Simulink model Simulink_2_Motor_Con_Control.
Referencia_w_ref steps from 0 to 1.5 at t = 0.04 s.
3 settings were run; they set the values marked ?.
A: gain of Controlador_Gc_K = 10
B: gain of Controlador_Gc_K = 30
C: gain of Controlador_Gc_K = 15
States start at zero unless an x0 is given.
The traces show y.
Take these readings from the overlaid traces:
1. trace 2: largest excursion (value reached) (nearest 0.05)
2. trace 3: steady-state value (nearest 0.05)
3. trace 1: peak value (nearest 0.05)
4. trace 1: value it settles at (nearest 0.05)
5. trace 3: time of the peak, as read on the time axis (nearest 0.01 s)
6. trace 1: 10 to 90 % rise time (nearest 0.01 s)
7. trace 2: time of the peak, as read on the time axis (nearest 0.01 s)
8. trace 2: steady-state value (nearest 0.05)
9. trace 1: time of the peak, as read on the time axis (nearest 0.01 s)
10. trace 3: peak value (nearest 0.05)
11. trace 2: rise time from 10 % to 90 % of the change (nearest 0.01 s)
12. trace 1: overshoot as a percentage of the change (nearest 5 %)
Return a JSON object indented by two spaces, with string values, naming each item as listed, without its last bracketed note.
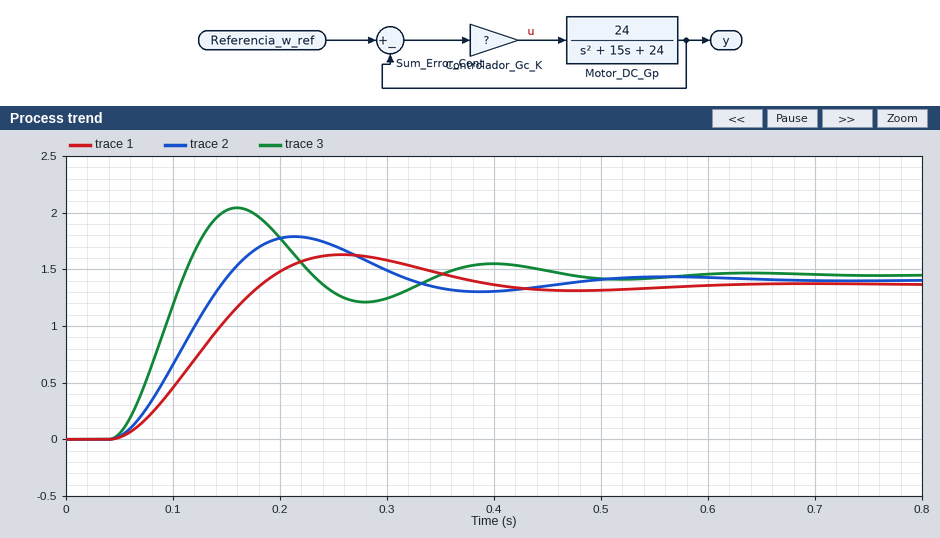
{
  "trace 2: largest excursion (value reached)": "1.80",
  "trace 3: steady-state value": "1.45",
  "trace 1: peak value": "1.65",
  "trace 1: value it settles at": "1.35",
  "trace 3: time of the peak, as read on the time axis": "0.16 s",
  "trace 1: 10 to 90 % rise time": "0.10 s",
  "trace 2: time of the peak, as read on the time axis": "0.21 s",
  "trace 2: steady-state value": "1.40",
  "trace 1: time of the peak, as read on the time axis": "0.26 s",
  "trace 3: peak value": "2.05",
  "trace 2: rise time from 10 % to 90 % of the change": "0.07 s",
  "trace 1: overshoot as a percentage of the change": "20 %"
}
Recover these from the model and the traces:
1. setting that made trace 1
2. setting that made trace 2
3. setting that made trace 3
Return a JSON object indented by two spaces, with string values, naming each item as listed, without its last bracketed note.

{
  "setting that made trace 1": "A",
  "setting that made trace 2": "C",
  "setting that made trace 3": "B"
}
